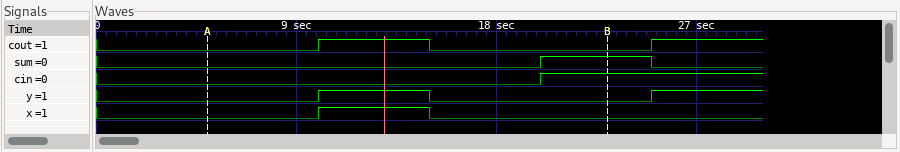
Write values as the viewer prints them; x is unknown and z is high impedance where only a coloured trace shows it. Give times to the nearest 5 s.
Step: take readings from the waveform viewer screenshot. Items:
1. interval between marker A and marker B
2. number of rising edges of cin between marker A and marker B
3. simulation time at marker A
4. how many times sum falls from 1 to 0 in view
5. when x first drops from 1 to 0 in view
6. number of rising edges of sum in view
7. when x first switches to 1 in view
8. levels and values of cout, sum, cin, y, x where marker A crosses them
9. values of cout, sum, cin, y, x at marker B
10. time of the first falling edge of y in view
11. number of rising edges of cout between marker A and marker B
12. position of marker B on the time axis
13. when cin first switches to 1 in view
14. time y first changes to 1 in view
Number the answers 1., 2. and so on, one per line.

1. 20 s
2. 1
3. 5 s
4. 1
5. 15 s
6. 1
7. 10 s
8. cout=0, sum=0, cin=0, y=0, x=0
9. cout=0, sum=1, cin=1, y=0, x=0
10. 15 s
11. 1
12. 25 s
13. 20 s
14. 10 s
